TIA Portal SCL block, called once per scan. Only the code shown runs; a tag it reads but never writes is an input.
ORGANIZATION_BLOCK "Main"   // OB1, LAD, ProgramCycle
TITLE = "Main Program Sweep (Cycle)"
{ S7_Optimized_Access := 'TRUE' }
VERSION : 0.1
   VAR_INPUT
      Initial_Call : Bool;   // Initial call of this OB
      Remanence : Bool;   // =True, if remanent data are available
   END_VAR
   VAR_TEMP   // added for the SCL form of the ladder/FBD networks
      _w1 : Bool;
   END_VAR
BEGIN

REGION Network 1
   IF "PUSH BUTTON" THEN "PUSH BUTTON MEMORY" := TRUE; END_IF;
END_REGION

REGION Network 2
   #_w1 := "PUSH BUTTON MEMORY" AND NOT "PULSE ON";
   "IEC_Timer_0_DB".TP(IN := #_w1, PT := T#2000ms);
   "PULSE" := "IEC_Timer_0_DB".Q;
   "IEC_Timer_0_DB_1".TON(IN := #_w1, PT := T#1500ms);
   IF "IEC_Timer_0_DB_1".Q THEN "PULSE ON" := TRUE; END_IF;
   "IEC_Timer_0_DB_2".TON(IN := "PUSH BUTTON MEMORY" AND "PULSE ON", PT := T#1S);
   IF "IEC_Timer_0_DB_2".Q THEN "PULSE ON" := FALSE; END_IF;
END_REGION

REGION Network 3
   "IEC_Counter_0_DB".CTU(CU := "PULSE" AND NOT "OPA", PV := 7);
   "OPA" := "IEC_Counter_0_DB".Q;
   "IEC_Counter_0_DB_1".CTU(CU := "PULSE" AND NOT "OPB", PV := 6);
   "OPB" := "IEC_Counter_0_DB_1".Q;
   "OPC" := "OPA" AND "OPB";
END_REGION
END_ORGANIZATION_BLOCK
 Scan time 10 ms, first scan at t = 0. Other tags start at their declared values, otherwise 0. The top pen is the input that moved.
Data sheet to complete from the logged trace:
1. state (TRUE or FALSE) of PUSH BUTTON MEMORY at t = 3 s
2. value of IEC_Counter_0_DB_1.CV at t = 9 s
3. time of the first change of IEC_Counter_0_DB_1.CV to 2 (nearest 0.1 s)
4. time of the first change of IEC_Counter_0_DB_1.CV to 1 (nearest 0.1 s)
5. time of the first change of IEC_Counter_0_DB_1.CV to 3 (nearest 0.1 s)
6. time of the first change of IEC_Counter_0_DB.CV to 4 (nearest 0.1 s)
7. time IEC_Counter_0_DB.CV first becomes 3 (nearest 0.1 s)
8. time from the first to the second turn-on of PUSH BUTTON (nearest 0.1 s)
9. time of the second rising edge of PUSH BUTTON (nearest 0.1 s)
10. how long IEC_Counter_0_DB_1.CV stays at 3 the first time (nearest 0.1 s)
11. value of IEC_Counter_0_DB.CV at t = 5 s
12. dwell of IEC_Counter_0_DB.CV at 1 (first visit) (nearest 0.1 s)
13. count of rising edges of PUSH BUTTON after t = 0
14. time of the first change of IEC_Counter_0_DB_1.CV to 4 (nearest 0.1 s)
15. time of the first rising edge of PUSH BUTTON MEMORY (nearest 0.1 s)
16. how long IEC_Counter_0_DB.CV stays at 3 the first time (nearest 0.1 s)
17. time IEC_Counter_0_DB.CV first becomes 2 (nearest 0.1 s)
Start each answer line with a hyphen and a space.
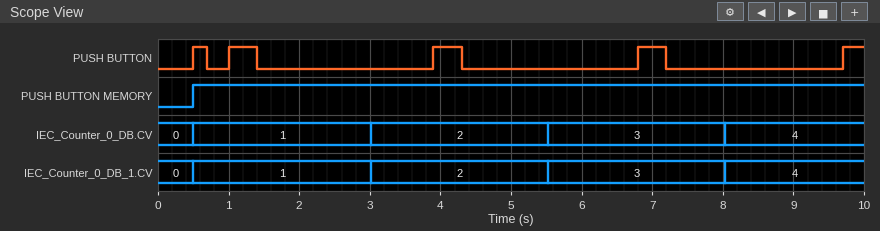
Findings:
- TRUE
- 4
- 3.0 s
- 0.5 s
- 5.5 s
- 8.0 s
- 5.5 s
- 0.5 s
- 1.0 s
- 2.5 s
- 2
- 2.5 s
- 5
- 8.0 s
- 0.5 s
- 2.5 s
- 3.0 s
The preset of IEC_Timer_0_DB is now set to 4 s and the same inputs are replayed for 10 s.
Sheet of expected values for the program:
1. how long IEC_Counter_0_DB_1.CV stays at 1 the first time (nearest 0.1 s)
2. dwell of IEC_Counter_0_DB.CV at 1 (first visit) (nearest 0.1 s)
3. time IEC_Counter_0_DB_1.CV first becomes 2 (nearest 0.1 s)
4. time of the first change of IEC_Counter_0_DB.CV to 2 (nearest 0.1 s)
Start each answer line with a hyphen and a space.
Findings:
- 5.0 s
- 5.0 s
- 5.5 s
- 5.5 s
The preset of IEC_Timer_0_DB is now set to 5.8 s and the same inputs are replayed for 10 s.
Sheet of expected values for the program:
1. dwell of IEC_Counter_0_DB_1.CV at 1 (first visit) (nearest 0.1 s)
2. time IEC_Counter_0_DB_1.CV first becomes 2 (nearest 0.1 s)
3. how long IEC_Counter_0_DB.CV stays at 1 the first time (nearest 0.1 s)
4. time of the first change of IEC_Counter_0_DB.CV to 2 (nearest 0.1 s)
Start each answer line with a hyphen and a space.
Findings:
- 7.5 s
- 8.0 s
- 7.5 s
- 8.0 s
